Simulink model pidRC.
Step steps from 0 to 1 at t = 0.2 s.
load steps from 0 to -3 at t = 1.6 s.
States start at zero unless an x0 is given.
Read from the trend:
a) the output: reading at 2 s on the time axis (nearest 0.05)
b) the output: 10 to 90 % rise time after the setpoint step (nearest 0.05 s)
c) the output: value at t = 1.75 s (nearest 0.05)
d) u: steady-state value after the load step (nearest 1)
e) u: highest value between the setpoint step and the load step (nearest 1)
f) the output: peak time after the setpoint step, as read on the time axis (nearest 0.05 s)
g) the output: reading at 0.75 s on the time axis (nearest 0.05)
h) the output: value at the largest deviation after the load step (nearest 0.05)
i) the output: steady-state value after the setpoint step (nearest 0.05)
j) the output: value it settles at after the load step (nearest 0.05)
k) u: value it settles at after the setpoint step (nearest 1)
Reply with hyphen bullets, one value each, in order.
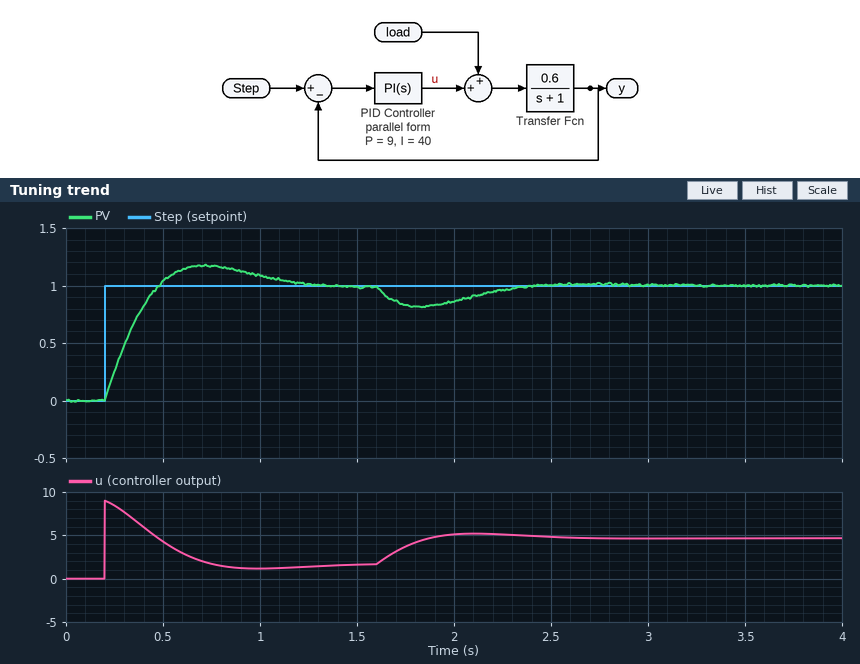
- 0.85
- 0.20 s
- 0.85
- 5
- 9
- 0.70 s
- 1.15
- 0.80
- 1.00
- 1.00
- 2
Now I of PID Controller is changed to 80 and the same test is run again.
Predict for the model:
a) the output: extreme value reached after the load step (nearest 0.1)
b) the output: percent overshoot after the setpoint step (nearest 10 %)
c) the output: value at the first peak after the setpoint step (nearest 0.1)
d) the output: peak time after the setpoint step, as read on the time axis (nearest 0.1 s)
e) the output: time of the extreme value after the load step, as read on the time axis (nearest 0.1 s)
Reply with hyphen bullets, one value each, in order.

- 0.9
- 30 %
- 1.3
- 0.6 s
- 1.8 s
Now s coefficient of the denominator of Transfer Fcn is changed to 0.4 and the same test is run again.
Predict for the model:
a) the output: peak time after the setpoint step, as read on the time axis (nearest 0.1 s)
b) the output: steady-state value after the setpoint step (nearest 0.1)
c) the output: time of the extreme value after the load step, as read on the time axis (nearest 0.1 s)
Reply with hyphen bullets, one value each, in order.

- 0.5 s
- 1.0
- 1.7 s
